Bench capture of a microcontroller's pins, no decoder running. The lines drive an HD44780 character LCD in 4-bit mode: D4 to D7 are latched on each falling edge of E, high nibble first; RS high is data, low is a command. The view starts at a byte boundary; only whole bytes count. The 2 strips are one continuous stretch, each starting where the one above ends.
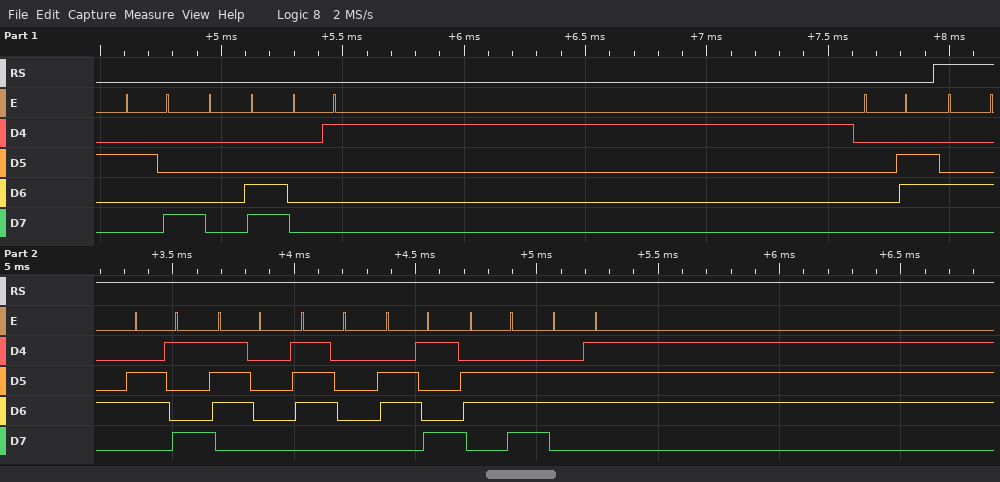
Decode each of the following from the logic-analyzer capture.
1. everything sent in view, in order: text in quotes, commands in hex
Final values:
0x28 0x0C 0x01 0x06 "Dipping"
